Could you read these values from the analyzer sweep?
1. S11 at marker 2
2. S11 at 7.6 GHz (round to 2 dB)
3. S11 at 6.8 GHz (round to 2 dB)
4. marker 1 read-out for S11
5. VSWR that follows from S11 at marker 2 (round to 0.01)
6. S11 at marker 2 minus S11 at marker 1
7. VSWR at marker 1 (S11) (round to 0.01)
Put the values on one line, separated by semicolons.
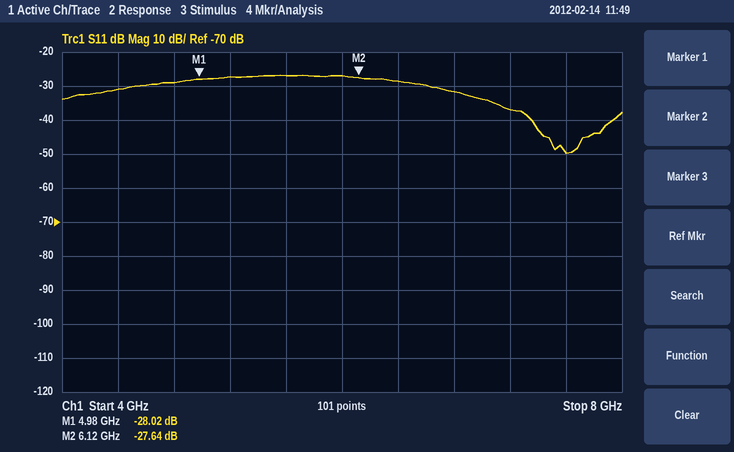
-27.64 dB; -50 dB; -32 dB; -28.02 dB; 1.09; 0.38 dB; 1.08
